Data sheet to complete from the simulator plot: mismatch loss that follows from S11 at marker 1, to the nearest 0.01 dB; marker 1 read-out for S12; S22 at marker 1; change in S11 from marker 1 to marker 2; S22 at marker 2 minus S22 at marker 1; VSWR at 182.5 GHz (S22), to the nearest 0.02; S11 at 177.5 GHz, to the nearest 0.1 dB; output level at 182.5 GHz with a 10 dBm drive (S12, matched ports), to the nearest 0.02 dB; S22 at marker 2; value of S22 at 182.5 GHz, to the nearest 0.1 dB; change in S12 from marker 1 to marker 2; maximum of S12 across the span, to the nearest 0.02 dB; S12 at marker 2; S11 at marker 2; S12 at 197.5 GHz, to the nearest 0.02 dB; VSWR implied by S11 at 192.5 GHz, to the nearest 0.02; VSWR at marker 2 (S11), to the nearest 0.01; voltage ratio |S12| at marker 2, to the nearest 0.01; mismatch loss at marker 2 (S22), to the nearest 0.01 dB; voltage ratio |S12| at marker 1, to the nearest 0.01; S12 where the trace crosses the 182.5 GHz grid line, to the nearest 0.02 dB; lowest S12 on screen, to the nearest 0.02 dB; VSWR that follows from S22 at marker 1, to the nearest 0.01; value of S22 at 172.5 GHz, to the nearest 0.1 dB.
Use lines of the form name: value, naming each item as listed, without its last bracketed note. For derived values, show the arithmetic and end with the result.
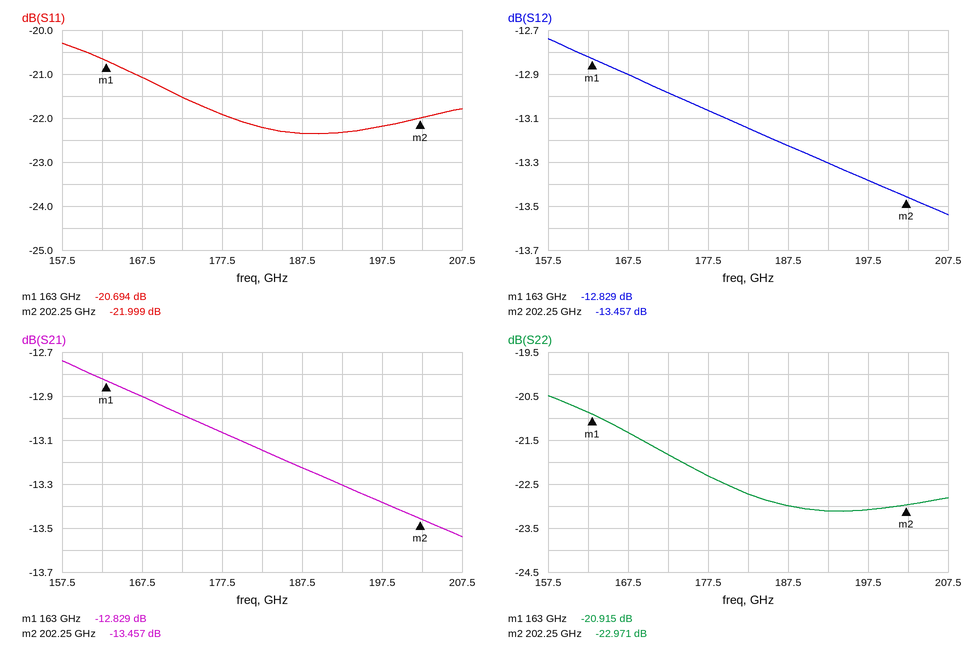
mismatch loss that follows from S11 at marker 1, to the nearest 0.01 dB: −10 log10(1 − 10^(-20.694/10)) ≈ 0.04 dB
marker 1 read-out for S12: -12.829 dB
S22 at marker 1: -20.915 dB
change in S11 from marker 1 to marker 2: -21.999 − (-20.694) = -1.305 dB
S22 at marker 2 minus S22 at marker 1: -22.971 − (-20.915) = -2.056 dB
VSWR at 182.5 GHz (S22), to the nearest 0.02: |Γ| = 10^(-22.7/20) = 0.0733; VSWR = (1 + 0.0733)/(1 − 0.0733) ≈ 1.16
S11 at 177.5 GHz, to the nearest 0.1 dB: -21.9 dB
output level at 182.5 GHz with a 10 dBm drive (S12, matched ports), to the nearest 0.02 dB: 10 dBm + (-13.14 dB) = -3.14 dBm
S22 at marker 2: -22.971 dB
value of S22 at 182.5 GHz, to the nearest 0.1 dB: -22.7 dB
change in S12 from marker 1 to marker 2: -13.457 − (-12.829) = -0.628 dB
maximum of S12 across the span, to the nearest 0.02 dB: -12.74 dB
S12 at marker 2: -13.457 dB
S11 at marker 2: -21.999 dB
S12 at 197.5 GHz, to the nearest 0.02 dB: -13.38 dB
VSWR implied by S11 at 192.5 GHz, to the nearest 0.02: |Γ| = 10^(-22.3/20) = 0.0767; VSWR = (1 + 0.0767)/(1 − 0.0767) ≈ 1.17, so 1.16 to the nearest 0.02
VSWR at marker 2 (S11), to the nearest 0.01: (1 + 0.0794)/(1 − 0.0794) ≈ 1.17
voltage ratio |S12| at marker 2, to the nearest 0.01: 10^(-13.457/20) ≈ 0.21
mismatch loss at marker 2 (S22), to the nearest 0.01 dB: −10 log10(1 − 10^(-22.971/10)) ≈ 0.02 dB
voltage ratio |S12| at marker 1, to the nearest 0.01: 10^(-12.829/20) ≈ 0.23
S12 where the trace crosses the 182.5 GHz grid line, to the nearest 0.02 dB: -13.14 dB
lowest S12 on screen, to the nearest 0.02 dB: -13.54 dB
VSWR that follows from S22 at marker 1, to the nearest 0.01: (1 + 0.0900)/(1 − 0.0900) ≈ 1.20
value of S22 at 172.5 GHz, to the nearest 0.1 dB: -21.8 dB
